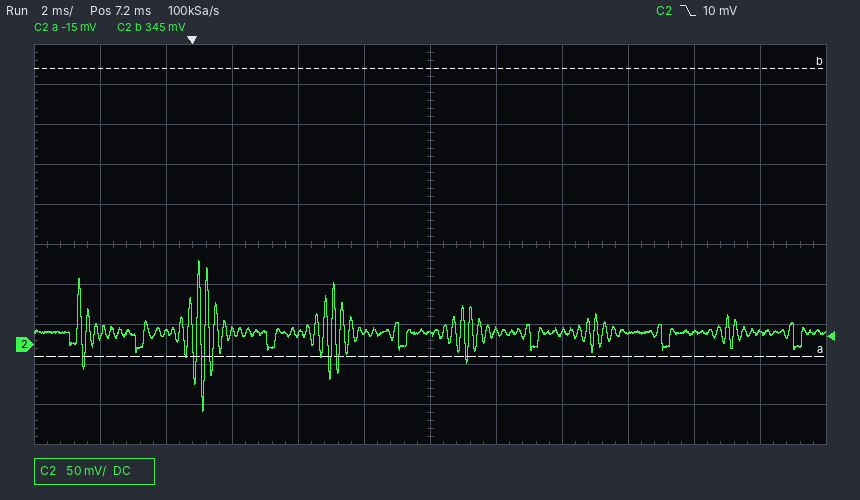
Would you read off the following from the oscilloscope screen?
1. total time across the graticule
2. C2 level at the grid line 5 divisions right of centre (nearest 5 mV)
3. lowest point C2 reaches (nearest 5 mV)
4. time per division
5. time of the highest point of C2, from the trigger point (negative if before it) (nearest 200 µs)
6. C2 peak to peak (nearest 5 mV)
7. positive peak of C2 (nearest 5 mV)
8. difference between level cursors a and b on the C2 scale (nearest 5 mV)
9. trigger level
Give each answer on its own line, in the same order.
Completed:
24 ms
15 mV
-85 mV
2 ms
+200 µs
190 mV
105 mV
360 mV
10 mV
